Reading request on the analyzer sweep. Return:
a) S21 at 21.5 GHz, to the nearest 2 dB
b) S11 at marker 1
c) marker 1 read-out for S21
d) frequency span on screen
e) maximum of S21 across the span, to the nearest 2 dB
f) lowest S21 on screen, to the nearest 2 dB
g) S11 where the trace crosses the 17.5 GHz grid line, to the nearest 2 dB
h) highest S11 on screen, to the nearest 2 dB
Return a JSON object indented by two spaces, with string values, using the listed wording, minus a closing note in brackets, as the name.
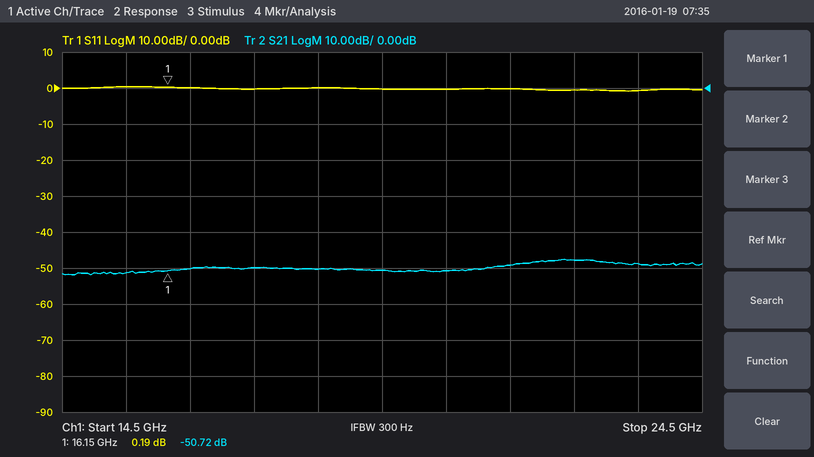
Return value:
{
  "S21 at 21.5 GHz, to the nearest 2 dB": "-50 dB",
  "S11 at marker 1": "0.19 dB",
  "marker 1 read-out for S21": "-50.72 dB",
  "frequency span on screen": "10 GHz",
  "maximum of S21 across the span, to the nearest 2 dB": "-48 dB",
  "lowest S21 on screen, to the nearest 2 dB": "-52 dB",
  "S11 where the trace crosses the 17.5 GHz grid line, to the nearest 2 dB": "0 dB",
  "highest S11 on screen, to the nearest 2 dB": "0 dB"
}
